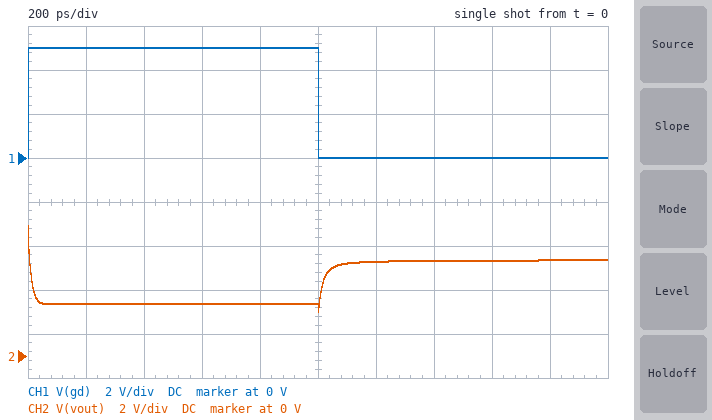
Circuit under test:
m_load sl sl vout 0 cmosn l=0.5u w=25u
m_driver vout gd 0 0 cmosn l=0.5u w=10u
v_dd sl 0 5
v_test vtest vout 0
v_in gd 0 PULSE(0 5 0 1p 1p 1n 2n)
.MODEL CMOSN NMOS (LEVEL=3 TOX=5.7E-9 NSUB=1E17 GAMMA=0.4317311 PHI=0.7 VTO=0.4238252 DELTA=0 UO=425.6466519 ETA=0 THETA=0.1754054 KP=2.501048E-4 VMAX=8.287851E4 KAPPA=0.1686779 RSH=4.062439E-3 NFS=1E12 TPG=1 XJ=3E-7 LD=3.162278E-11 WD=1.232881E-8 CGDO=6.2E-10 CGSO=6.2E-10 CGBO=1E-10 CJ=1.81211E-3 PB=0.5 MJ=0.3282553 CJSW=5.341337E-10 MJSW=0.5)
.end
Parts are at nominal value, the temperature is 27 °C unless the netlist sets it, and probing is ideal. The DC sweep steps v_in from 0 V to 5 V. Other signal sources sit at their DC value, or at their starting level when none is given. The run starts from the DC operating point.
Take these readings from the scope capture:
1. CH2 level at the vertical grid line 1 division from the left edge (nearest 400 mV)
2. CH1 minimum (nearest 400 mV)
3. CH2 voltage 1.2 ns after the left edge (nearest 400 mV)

2.4 V
0 V
4.4 V
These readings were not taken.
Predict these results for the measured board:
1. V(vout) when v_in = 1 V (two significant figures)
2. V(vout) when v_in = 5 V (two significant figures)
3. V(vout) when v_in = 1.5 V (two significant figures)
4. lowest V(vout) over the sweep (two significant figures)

4.0 V
2.3 V
3.7 V
2.3 V
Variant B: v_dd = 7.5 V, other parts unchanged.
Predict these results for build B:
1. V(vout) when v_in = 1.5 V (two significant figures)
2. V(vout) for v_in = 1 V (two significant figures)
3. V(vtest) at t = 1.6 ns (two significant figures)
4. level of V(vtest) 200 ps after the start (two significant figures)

6.1 V
6.4 V
6.8 V
4.6 V
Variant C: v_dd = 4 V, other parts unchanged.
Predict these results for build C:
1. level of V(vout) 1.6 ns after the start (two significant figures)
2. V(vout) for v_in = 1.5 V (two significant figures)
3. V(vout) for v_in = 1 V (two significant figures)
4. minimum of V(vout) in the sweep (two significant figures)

3.4 V
2.8 V
3.0 V
1.5 V
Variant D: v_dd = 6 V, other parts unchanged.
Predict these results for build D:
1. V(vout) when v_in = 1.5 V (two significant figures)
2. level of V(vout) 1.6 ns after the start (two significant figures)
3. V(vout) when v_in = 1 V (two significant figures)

4.7 V
5.3 V
4.9 V
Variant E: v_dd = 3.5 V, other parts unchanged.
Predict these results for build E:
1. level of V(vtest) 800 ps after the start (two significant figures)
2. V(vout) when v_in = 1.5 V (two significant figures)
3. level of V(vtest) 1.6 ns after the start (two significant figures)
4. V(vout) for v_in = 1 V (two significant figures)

1.1 V
2.3 V
2.9 V
2.5 V
